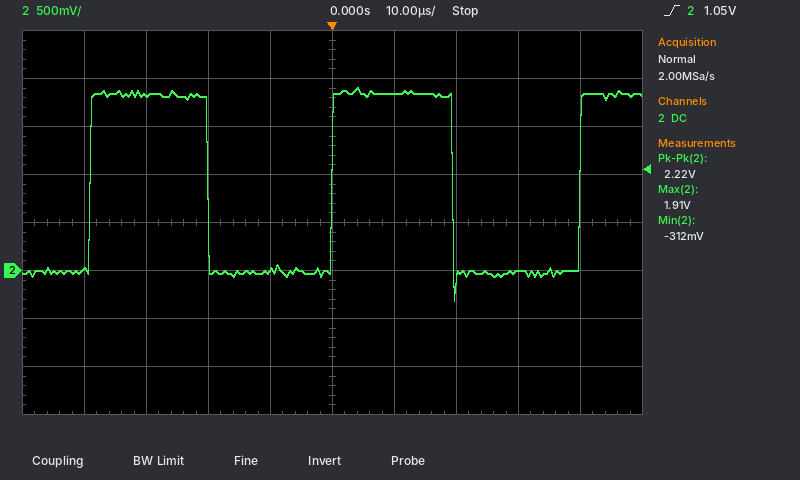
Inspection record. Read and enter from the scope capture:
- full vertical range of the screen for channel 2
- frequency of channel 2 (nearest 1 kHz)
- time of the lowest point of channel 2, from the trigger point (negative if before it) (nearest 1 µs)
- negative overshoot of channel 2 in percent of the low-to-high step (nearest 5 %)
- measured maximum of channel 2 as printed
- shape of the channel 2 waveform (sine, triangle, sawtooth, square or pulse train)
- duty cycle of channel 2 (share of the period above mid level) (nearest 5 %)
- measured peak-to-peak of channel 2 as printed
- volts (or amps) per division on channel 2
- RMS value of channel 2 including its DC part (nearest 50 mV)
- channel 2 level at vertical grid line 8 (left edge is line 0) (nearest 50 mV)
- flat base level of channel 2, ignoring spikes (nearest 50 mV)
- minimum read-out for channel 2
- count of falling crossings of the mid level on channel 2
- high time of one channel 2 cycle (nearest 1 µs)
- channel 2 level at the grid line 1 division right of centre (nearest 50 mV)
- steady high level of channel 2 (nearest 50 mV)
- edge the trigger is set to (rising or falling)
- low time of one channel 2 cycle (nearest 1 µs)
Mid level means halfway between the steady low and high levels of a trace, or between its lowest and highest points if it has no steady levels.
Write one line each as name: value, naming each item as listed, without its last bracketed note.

full vertical range of the screen for channel 2: 4 V
frequency of channel 2: 25 kHz
time of the lowest point of channel 2, from the trigger point (negative if before it): +20 µs
negative overshoot of channel 2 in percent of the low-to-high step: 15 %
measured maximum of channel 2 as printed: 1.91 V
shape of the channel 2 waveform: square
duty cycle of channel 2 (share of the period above mid level): 50 %
measured peak-to-peak of channel 2 as printed: 2.22 V
volts (or amps) per division on channel 2: 500 mV
RMS value of channel 2 including its DC part: 1.30 V
channel 2 level at vertical grid line 8 (left edge is line 0): 0 mV
flat base level of channel 2, ignoring spikes: 0 mV
minimum read-out for channel 2: -312 mV
count of falling crossings of the mid level on channel 2: 2
high time of one channel 2 cycle: 19 µs
channel 2 level at the grid line 1 division right of centre: 1.85 V
steady high level of channel 2: 1.85 V
edge the trigger is set to: rising
low time of one channel 2 cycle: 20 µs
